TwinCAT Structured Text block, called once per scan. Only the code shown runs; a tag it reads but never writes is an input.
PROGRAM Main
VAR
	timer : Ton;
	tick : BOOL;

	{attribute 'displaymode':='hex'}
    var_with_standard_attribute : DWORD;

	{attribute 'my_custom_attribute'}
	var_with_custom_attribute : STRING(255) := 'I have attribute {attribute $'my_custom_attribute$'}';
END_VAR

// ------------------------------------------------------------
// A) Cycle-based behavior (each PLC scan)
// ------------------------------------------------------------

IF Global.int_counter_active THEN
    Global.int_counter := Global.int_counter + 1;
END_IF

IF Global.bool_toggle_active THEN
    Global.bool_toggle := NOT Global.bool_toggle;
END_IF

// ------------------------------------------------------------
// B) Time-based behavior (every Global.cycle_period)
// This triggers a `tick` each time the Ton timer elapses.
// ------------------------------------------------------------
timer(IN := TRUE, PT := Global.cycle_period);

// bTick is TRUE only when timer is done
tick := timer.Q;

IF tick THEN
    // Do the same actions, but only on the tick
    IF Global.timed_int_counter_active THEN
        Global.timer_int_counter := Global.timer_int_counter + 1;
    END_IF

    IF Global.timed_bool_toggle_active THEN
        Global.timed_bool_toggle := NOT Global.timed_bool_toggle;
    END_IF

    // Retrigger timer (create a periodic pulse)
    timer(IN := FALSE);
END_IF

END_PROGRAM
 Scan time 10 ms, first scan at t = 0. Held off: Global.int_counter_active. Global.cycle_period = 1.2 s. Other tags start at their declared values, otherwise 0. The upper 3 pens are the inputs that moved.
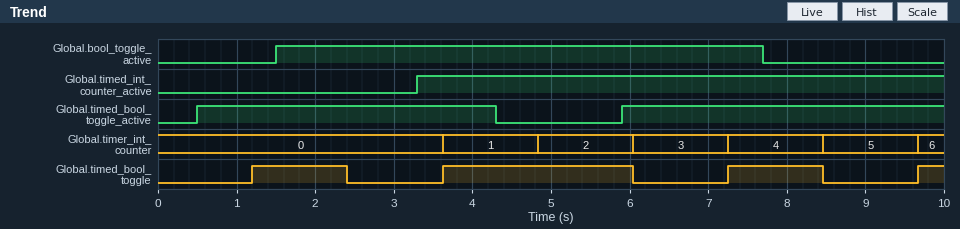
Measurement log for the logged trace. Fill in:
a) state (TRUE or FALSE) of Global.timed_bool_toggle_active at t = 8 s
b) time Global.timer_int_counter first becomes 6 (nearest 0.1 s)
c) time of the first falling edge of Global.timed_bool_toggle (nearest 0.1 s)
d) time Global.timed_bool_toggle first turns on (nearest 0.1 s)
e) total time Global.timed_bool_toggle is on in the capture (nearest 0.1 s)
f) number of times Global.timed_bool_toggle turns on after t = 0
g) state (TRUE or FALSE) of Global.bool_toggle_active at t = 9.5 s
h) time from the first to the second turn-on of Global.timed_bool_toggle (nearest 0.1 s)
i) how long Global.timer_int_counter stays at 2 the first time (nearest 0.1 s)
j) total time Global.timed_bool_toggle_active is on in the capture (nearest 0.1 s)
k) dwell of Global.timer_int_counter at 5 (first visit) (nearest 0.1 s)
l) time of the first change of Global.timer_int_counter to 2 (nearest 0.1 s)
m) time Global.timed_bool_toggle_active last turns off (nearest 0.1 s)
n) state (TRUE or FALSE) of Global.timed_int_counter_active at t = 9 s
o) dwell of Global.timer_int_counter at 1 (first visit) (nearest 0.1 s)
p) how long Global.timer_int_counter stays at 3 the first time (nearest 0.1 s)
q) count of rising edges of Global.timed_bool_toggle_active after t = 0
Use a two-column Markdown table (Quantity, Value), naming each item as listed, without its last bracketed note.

| Quantity | Value |
|---|---|
| state (TRUE or FALSE) of Global.timed_bool_toggle_active at t = 8 s | TRUE |
| time Global.timer_int_counter first becomes 6 | 9.7 s |
| time of the first falling edge of Global.timed_bool_toggle | 2.4 s |
| time Global.timed_bool_toggle first turns on | 1.2 s |
| total time Global.timed_bool_toggle is on in the capture | 5.2 s |
| number of times Global.timed_bool_toggle turns on after t = 0 | 4 |
| state (TRUE or FALSE) of Global.bool_toggle_active at t = 9.5 s | FALSE |
| time from the first to the second turn-on of Global.timed_bool_toggle | 2.4 s |
| how long Global.timer_int_counter stays at 2 the first time | 1.2 s |
| total time Global.timed_bool_toggle_active is on in the capture | 7.9 s |
| dwell of Global.timer_int_counter at 5 (first visit) | 1.2 s |
| time of the first change of Global.timer_int_counter to 2 | 4.8 s |
| time Global.timed_bool_toggle_active last turns off | 4.3 s |
| state (TRUE or FALSE) of Global.timed_int_counter_active at t = 9 s | TRUE |
| dwell of Global.timer_int_counter at 1 (first visit) | 1.2 s |
| how long Global.timer_int_counter stays at 3 the first time | 1.2 s |
| count of rising edges of Global.timed_bool_toggle_active after t = 0 | 2 |
